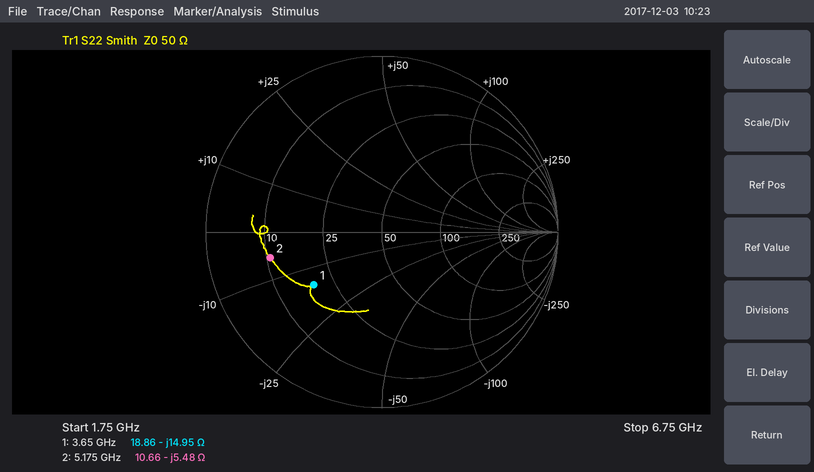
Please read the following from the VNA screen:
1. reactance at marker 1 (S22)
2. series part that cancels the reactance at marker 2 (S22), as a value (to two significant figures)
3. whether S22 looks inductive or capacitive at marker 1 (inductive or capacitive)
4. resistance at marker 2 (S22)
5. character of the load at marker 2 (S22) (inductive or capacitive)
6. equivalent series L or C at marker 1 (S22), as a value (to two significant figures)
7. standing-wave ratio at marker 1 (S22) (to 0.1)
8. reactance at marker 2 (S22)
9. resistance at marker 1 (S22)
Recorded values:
-14.95 Ω
170 pH
capacitive
10.66 Ω
capacitive
2.9 pF
2.9
-5.48 Ω
18.86 Ω
